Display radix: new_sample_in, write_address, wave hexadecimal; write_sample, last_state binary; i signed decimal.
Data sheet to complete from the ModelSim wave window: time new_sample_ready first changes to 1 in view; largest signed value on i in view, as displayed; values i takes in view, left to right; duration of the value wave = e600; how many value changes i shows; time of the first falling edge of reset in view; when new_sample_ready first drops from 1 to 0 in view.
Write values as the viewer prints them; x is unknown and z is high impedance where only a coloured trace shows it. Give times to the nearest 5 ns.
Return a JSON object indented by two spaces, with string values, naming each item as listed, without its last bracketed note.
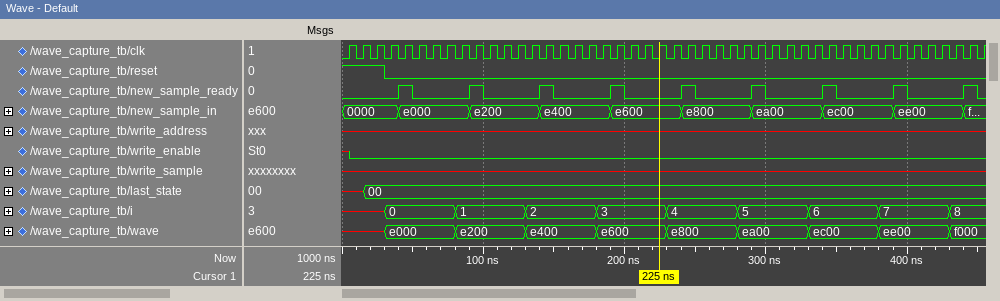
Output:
{
  "time new_sample_ready first changes to 1 in view": "40 ns",
  "largest signed value on i in view, as displayed": "8",
  "values i takes in view, left to right": "x, 0, 1, 2, 3, 4, 5, 6, 7, 8",
  "duration of the value wave = e600": "50 ns",
  "how many value changes i shows": "9",
  "time of the first falling edge of reset in view": "30 ns",
  "when new_sample_ready first drops from 1 to 0 in view": "50 ns"
}
